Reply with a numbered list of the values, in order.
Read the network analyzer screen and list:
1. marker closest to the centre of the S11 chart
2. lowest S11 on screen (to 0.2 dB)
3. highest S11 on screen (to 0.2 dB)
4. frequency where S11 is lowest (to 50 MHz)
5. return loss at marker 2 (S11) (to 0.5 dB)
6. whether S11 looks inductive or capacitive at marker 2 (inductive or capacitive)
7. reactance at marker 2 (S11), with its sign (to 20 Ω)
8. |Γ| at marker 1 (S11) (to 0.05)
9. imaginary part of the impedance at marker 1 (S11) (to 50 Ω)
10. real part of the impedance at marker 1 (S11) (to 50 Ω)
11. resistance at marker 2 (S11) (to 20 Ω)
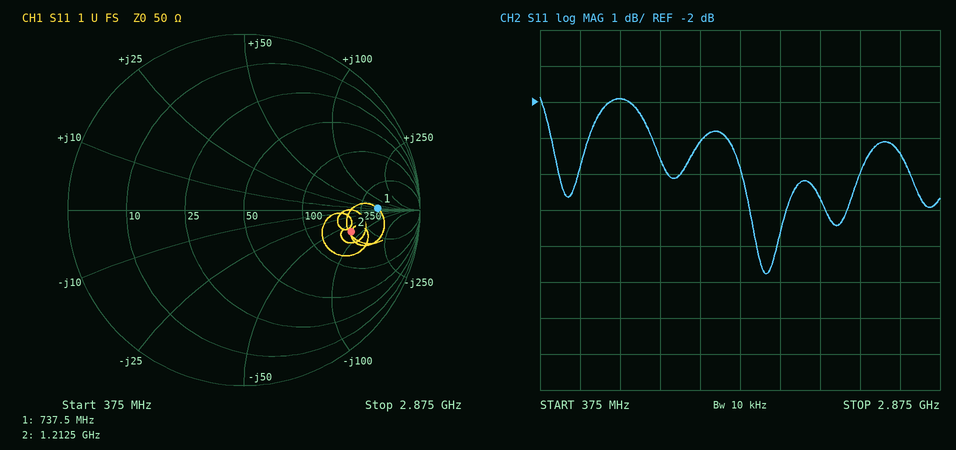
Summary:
1. marker 2
2. -6.8 dB
3. -1.8 dB
4. 1.80 GHz
5. 4.0 dB
6. capacitive
7. -80 Ω
8. 0.75
9. 0 Ω
10. 350 Ω
11. 180 Ω
